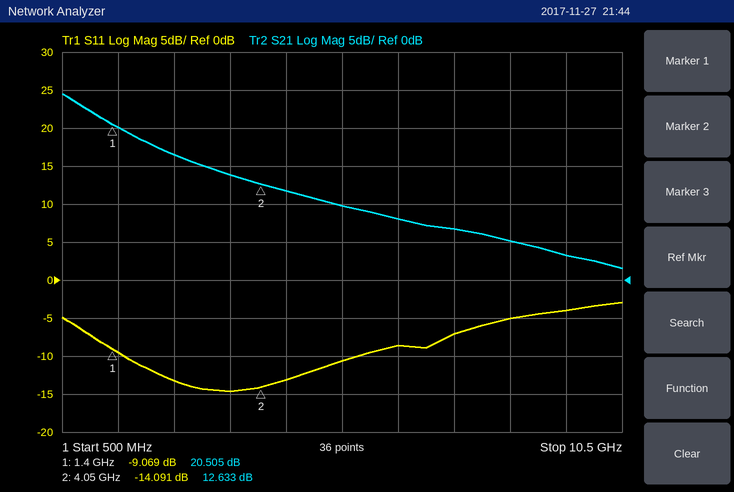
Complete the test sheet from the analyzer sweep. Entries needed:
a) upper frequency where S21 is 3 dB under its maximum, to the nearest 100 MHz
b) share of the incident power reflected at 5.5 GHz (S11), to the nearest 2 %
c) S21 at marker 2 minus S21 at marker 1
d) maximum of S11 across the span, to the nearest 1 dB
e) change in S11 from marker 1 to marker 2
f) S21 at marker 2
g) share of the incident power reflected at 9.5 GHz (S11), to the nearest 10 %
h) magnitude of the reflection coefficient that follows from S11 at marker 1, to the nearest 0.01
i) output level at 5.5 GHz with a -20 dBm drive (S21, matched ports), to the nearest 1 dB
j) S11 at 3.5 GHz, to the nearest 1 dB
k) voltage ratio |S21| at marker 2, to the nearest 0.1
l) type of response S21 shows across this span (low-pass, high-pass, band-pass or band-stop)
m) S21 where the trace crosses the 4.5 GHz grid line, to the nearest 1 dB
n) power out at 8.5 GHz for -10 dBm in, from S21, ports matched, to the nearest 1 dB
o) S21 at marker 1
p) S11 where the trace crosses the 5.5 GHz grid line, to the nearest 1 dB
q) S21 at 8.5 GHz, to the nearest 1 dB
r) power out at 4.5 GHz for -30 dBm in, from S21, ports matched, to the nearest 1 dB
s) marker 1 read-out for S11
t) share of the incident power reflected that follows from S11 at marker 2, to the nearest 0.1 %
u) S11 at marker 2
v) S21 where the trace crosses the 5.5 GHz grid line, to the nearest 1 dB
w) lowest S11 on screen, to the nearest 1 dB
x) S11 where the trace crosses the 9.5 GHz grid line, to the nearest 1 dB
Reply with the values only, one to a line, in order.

1.2 GHz
8 %
-7.872 dB
-3 dB
-5.022 dB
12.633 dB
40 %
0.35
-10 dBm
-15 dB
4.3
low-pass
12 dB
-5 dBm
20.505 dB
-11 dB
5 dB
-18 dBm
-9.069 dB
3.9 %
-14.091 dB
10 dB
-15 dB
-4 dB
